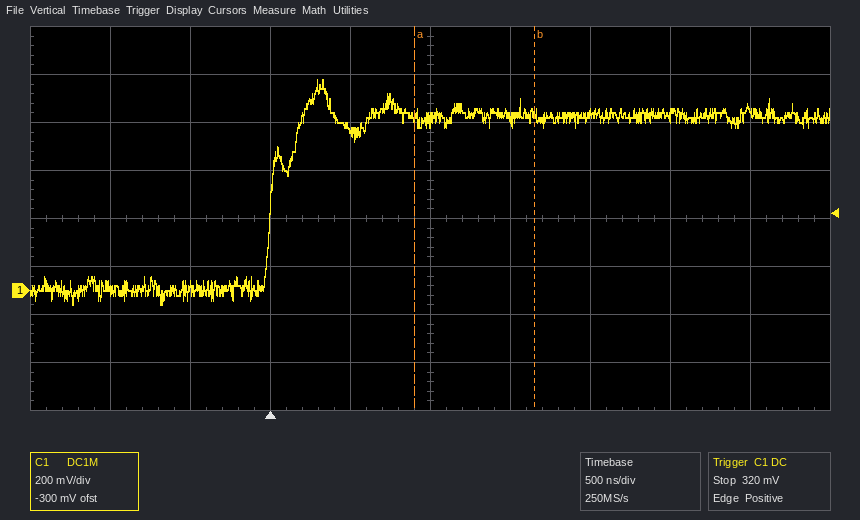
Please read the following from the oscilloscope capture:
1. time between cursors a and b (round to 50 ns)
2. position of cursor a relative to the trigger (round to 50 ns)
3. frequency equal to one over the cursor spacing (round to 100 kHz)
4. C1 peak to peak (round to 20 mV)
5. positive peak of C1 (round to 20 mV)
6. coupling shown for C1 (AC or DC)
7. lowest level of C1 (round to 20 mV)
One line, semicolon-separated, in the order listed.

750 ns; +900 ns; 1.3 MHz; 940 mV; 880 mV; DC; -60 mV
